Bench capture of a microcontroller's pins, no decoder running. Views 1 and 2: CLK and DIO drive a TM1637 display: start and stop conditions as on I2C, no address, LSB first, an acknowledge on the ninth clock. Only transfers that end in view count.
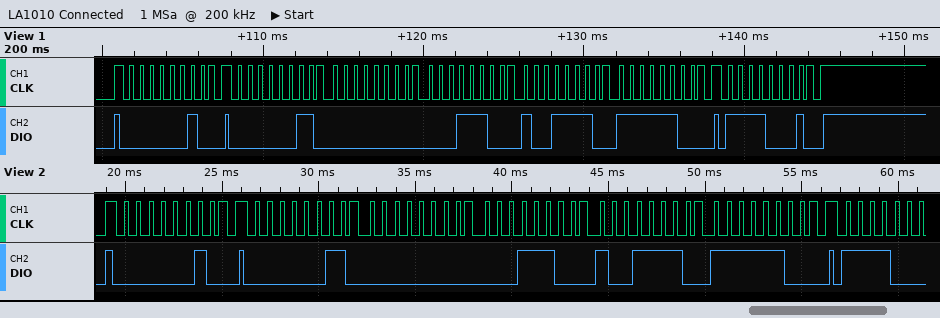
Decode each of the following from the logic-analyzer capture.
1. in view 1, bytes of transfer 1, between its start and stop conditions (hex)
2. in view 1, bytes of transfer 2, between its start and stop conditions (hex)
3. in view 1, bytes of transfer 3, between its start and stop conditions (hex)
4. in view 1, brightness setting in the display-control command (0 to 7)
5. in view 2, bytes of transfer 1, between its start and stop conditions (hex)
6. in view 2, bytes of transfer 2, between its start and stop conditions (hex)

40
C0 00 38 79 3F
8F
7
40
C0 00 38 79 3F
